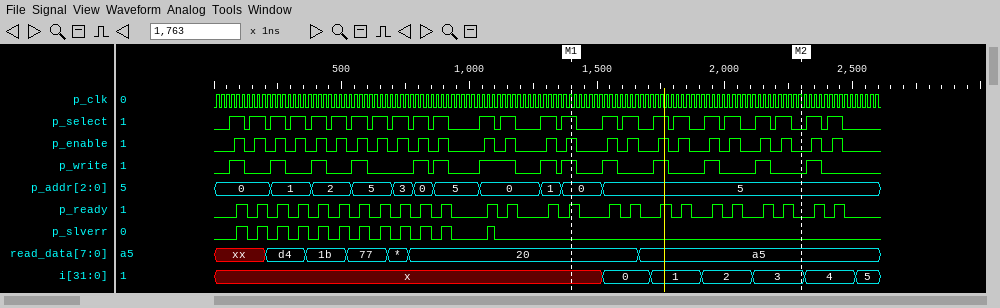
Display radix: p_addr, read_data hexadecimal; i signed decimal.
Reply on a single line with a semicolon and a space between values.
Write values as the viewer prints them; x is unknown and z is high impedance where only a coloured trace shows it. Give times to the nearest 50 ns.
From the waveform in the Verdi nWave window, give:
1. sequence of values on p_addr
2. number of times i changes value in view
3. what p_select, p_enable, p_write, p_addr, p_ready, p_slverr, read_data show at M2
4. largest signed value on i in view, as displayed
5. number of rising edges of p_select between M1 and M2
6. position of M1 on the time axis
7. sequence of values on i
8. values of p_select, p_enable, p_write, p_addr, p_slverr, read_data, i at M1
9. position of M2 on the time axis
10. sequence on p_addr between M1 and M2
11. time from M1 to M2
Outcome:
0, 1, 2, 5, 3, 0, 5, 0, 1, 0, 5; 6; p_select=0, p_enable=0, p_write=0, p_addr=5, p_ready=0, p_slverr=0, read_data=a5; 5; 8; 1400 ns; x, 0, 1, 2, 3, 4, 5; p_select=1, p_enable=1, p_write=1, p_addr=0, p_slverr=0, read_data=20, i=x; 2300 ns; 0, 5; 900 ns
